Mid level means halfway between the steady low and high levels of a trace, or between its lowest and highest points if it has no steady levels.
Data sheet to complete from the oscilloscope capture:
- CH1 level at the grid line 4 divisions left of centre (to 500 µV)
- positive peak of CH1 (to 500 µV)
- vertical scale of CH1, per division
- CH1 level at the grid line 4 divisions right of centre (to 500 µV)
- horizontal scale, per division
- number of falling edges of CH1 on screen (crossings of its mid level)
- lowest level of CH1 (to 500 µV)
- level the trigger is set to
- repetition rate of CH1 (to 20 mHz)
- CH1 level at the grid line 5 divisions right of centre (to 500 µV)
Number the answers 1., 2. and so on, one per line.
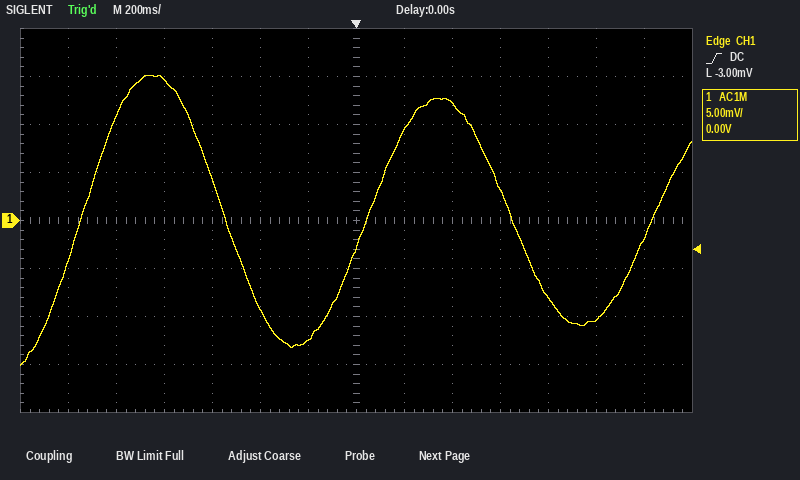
1. 14.5 mV
2. 15.0 mV
3. 5 mV
4. -8.0 mV
5. 200 ms
6. 2
7. -15.0 mV
8. -3.00 mV
9. 840 mHz
10. -10.5 mV
